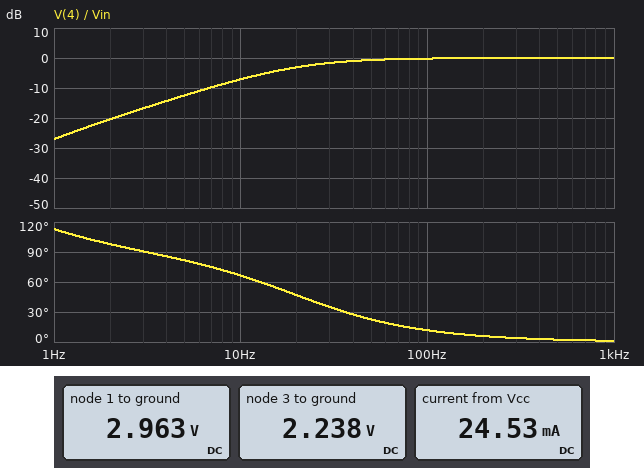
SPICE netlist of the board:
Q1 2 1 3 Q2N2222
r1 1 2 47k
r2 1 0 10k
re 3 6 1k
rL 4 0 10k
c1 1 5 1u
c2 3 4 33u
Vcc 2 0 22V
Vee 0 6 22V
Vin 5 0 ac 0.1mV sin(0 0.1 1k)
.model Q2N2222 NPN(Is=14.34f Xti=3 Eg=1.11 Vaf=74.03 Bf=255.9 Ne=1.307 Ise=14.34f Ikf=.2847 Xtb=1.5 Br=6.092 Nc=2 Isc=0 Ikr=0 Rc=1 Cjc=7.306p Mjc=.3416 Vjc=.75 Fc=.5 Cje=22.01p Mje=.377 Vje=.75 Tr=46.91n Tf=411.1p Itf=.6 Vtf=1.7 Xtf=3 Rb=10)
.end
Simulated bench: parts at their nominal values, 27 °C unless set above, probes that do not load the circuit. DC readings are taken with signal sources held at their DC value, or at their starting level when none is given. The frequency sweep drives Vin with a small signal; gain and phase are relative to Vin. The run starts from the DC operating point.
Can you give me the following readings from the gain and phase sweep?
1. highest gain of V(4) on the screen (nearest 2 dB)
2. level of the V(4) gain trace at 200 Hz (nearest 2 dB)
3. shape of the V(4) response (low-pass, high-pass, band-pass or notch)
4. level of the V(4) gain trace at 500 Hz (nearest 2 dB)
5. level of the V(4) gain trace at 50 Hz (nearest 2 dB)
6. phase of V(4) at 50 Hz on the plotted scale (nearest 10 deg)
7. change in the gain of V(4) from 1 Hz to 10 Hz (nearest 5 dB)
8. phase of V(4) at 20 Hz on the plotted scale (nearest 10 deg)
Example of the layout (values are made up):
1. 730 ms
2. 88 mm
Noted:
1. 0 dB
2. 0 dB
3. high-pass
4. 0 dB
5. 0 dB
6. 20 deg
7. 20 dB
8. 50 deg
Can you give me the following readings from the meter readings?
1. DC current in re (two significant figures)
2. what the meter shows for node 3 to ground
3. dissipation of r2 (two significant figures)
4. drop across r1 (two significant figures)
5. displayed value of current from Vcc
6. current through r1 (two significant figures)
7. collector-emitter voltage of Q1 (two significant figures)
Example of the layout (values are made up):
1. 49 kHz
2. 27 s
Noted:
1. 24 mA
2. 2.238 V
3. 880 µW
4. 19 V
5. 24.53 mA
6. 410 µA
7. 20 V
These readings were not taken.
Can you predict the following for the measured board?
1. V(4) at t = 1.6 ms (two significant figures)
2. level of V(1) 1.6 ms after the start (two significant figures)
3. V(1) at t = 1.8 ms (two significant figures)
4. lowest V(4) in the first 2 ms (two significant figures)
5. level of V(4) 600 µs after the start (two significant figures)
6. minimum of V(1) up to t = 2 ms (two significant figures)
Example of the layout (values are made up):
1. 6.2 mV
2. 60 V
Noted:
1. -62 mV
2. 2.9 V
3. 2.9 V
4. -100 mV
5. -62 mV
6. 2.9 V
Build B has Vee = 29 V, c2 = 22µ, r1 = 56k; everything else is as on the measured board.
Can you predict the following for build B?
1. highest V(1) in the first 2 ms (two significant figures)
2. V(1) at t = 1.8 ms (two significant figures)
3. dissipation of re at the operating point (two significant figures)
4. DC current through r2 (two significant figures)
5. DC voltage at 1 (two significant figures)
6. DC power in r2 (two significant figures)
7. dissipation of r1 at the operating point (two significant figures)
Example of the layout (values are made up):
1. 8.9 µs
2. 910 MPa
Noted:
1. 2.3 V
2. 2.1 V
3. 930 mW
4. 220 µA
5. 2.2 V
6. 480 µW
7. 7.0 mW
